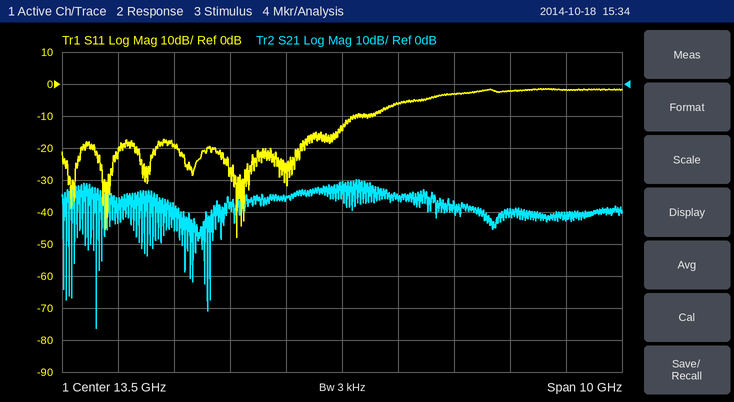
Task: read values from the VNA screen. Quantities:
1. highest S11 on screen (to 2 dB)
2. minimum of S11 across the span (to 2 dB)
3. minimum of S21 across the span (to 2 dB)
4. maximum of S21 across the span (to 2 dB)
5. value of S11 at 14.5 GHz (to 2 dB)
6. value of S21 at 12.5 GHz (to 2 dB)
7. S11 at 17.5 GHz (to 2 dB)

-2 dB
-48 dB
-76 dB
-30 dB
-6 dB
-36 dB
-2 dB
